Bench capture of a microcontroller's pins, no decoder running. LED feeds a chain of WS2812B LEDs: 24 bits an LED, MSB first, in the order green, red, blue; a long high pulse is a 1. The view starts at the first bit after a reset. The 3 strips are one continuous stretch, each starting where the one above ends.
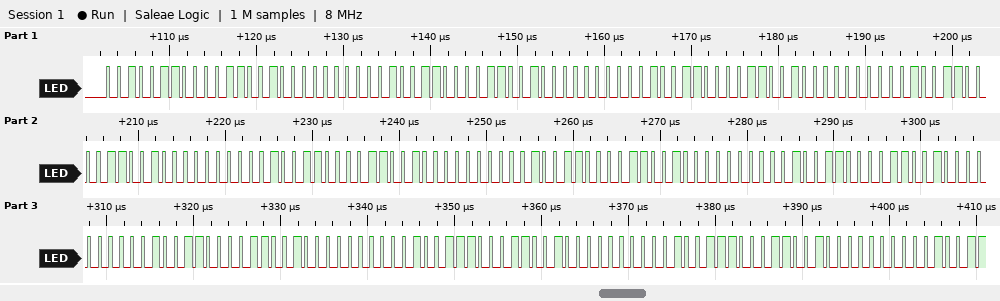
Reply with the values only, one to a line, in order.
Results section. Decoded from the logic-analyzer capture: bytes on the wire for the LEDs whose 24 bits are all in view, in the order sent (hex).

26 19 00 26 19 00 26 19 00 26 19 00 26 19 00 26 19 00 26 19 00 26 19 00 27 19 00 27 19 00
